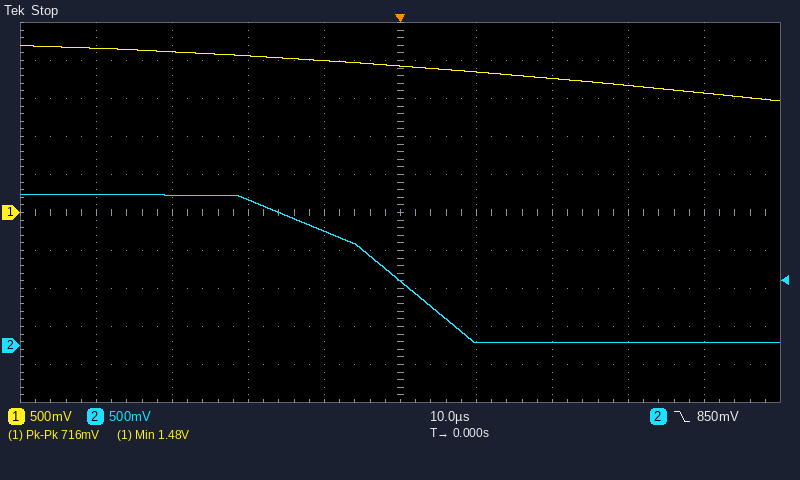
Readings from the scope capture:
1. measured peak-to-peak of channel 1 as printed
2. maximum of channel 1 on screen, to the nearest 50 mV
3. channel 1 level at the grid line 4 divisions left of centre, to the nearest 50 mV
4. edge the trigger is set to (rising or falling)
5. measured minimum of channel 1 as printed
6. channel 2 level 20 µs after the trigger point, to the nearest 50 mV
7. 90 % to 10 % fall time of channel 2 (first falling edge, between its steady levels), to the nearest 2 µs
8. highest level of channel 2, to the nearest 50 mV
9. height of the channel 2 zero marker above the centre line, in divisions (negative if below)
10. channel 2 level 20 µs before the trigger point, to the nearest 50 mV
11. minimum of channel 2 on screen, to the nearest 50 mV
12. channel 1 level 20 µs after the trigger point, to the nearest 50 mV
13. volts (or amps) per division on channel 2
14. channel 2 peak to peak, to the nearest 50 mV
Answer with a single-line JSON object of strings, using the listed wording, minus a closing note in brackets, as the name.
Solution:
{"measured peak-to-peak of channel 1 as printed": "716 mV", "maximum of channel 1 on screen, to the nearest 50 mV": "2.20 V", "channel 1 level at the grid line 4 divisions left of centre, to the nearest 50 mV": "2.15 V", "edge the trigger is set to": "falling", "measured minimum of channel 1 as printed": "1.48 V", "channel 2 level 20 µs after the trigger point, to the nearest 50 mV": "50 mV", "90 % to 10 % fall time of channel 2 (first falling edge, between its steady levels), to the nearest 2 µs": "24 µs", "highest level of channel 2, to the nearest 50 mV": "2.00 V", "height of the channel 2 zero marker above the centre line, in divisions": "-3.5 div", "channel 2 level 20 µs before the trigger point, to the nearest 50 mV": "1.90 V", "minimum of channel 2 on screen, to the nearest 50 mV": "50 mV", "channel 1 level 20 µs after the trigger point, to the nearest 50 mV": "1.75 V", "volts (or amps) per division on channel 2": "500 mV", "channel 2 peak to peak, to the nearest 50 mV": "1.95 V"}
